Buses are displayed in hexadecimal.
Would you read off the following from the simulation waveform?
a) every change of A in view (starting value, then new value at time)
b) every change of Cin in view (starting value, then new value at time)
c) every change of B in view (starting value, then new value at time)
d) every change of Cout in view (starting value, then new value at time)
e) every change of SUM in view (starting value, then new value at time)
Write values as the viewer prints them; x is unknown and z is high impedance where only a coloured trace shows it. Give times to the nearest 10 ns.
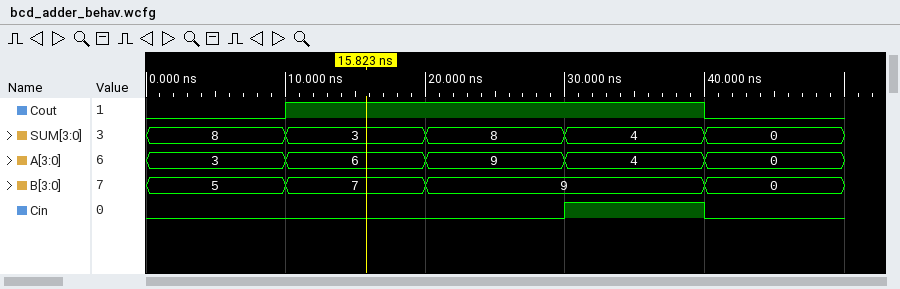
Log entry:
3, 6 at 10 ns, 9 at 20 ns, 4 at 30 ns, 0 at 40 ns
0, 1 at 30 ns, 0 at 40 ns
5, 7 at 10 ns, 9 at 20 ns, 0 at 40 ns
0, 1 at 10 ns, 0 at 40 ns
8, 3 at 10 ns, 8 at 20 ns, 4 at 30 ns, 0 at 40 ns
